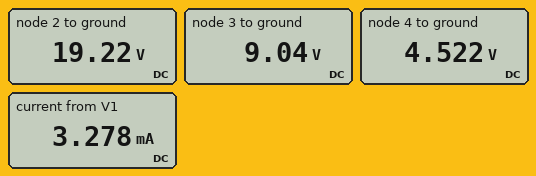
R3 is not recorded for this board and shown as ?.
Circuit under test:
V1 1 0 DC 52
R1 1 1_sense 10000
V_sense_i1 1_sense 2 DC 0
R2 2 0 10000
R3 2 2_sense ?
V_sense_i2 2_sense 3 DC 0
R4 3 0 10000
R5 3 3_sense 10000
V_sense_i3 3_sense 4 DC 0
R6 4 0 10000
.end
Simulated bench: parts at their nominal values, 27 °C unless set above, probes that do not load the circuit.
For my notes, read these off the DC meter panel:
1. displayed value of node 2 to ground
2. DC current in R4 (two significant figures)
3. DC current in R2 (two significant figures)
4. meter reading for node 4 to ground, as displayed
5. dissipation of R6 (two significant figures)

19.22 V
900 µA
1.9 mA
4.522 V
2.0 mW
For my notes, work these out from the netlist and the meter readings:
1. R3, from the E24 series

7.5 kΩ
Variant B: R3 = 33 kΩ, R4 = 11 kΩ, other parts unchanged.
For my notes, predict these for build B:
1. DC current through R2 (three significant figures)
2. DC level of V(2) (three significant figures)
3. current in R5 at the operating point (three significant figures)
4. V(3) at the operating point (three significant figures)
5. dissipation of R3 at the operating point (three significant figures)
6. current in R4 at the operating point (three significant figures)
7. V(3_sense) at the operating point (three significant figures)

2.31 mA
23.1 V
205 µA
4.09 V
11.0 mW
372 µA
2.05 V
